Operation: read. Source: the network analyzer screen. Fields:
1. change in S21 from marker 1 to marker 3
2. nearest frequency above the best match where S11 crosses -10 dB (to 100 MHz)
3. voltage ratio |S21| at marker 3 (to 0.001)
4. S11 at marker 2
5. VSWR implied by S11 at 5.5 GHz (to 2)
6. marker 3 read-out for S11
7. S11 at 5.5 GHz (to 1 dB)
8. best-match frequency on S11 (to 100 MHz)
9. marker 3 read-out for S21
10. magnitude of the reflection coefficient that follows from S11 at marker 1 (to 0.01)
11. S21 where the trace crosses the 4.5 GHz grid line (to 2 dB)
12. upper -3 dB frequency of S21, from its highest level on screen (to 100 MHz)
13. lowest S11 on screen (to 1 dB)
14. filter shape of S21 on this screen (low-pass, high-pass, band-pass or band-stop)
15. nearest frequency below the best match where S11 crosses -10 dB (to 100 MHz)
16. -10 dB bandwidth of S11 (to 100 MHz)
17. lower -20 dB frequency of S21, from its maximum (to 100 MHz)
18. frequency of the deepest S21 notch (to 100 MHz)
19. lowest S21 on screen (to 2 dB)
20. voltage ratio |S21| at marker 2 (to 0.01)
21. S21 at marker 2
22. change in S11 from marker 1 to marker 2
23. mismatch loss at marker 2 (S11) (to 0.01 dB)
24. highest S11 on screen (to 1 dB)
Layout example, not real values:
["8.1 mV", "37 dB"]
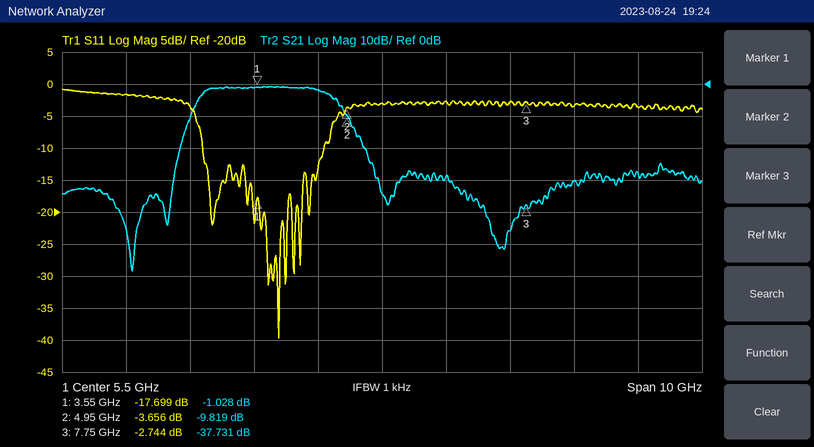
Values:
["-36.703 dB", "4.6 GHz", "0.013", "-3.656 dB", "6", "-2.744 dB", "-3 dB", "3.9 GHz", "-37.731 dB", "0.13", "-2 dB", "4.7 GHz", "-40 dB", "band-pass", "2.7 GHz", "1.9 GHz", "2.3 GHz", "1.6 GHz", "-58 dB", "0.32", "-9.819 dB", "14.043 dB", "2.45 dB", "-1 dB"]
